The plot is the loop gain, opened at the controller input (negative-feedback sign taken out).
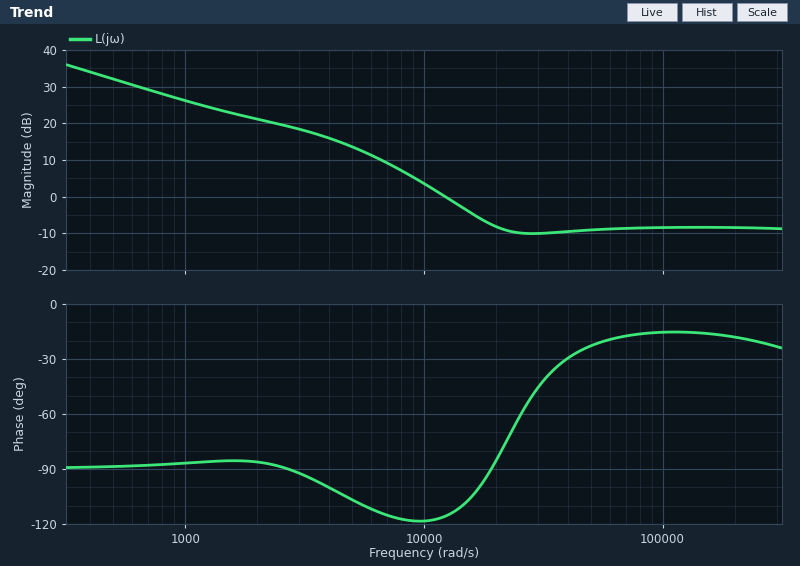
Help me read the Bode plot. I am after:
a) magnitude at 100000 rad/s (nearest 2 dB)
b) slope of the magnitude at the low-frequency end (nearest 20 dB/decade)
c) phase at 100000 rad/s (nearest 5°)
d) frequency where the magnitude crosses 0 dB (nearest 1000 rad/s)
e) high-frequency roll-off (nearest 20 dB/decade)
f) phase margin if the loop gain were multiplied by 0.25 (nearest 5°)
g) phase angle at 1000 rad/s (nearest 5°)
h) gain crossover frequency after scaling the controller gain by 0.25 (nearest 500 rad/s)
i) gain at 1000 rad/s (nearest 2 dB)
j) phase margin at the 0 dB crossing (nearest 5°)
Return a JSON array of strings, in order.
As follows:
["-8 dB", "-20 dB/decade", "-15°", "12000 rad/s", "0 dB/decade", "70°", "-85°", "5500 rad/s", "26 dB", "65°"]
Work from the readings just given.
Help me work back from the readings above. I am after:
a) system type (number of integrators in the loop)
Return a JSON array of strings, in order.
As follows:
["1"]
